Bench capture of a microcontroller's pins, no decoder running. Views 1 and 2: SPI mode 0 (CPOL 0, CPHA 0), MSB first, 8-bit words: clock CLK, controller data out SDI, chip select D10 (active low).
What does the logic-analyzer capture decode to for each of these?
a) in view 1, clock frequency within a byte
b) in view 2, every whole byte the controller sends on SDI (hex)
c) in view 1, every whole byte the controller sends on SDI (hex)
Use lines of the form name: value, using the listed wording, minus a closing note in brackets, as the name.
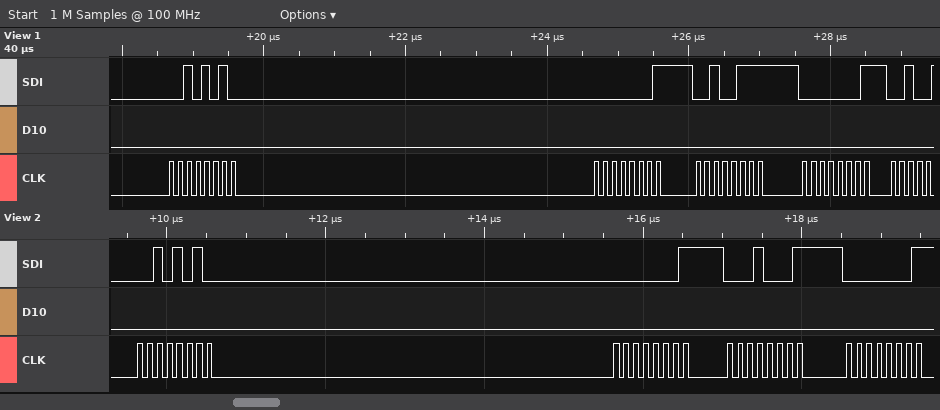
in view 1, clock frequency within a byte: 8 MHz
in view 2, every whole byte the controller sends on SDI: 0x2A 0x01 0x11 0x01
in view 1, every whole byte the controller sends on SDI: 2A 01 27 01
